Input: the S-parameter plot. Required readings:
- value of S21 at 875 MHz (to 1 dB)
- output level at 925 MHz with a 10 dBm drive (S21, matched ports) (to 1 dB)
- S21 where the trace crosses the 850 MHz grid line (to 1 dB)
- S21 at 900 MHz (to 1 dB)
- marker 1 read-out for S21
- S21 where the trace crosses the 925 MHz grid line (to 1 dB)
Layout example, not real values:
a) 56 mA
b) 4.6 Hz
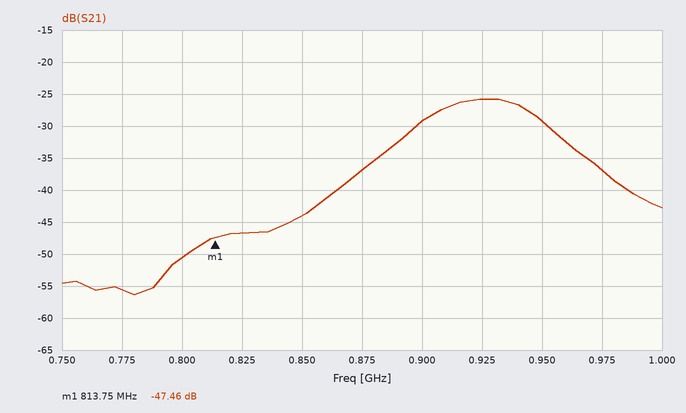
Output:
a) -37 dB
b) -16 dBm
c) -44 dB
d) -29 dB
e) -47.46 dB
f) -26 dB
